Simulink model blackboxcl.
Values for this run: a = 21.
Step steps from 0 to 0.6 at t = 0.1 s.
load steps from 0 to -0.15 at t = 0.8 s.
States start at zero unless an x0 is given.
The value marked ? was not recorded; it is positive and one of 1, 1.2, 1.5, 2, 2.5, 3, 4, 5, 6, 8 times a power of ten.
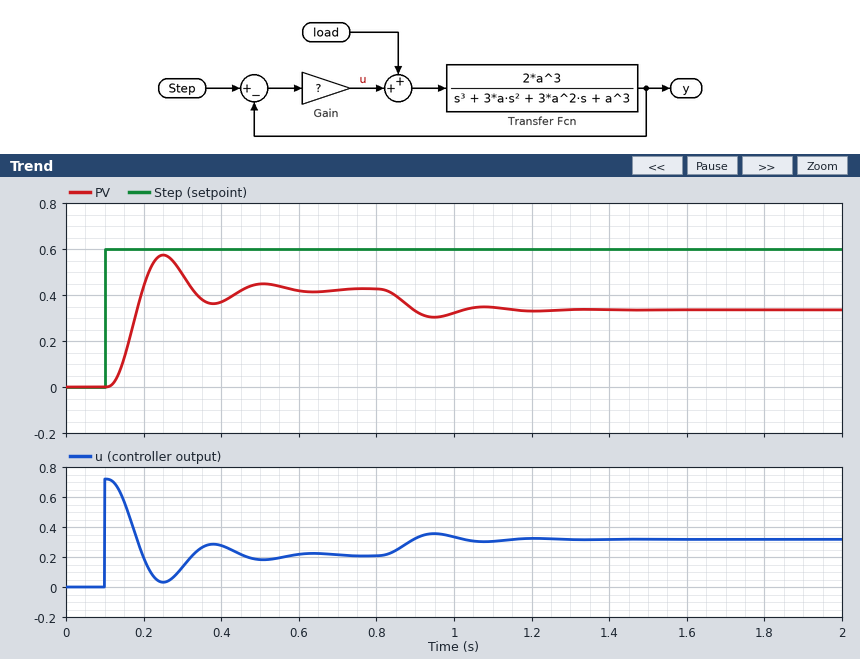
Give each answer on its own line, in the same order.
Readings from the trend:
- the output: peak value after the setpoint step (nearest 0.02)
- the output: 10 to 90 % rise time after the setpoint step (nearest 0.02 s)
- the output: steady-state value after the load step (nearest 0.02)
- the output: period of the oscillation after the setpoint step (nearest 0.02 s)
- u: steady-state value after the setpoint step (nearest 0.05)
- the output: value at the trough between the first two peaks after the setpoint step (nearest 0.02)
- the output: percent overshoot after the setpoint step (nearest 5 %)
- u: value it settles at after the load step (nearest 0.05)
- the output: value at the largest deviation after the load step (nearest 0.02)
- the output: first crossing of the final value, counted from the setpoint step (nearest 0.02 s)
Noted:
0.58
0.06 s
0.34
0.26 s
0.20
0.36
35 %
0.30
0.30
0.10 s
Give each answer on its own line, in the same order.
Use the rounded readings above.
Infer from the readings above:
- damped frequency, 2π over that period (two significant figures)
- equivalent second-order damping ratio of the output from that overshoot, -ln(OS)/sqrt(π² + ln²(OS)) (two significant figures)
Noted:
24 rad/s
0.32
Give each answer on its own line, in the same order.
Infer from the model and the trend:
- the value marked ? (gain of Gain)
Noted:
1.2
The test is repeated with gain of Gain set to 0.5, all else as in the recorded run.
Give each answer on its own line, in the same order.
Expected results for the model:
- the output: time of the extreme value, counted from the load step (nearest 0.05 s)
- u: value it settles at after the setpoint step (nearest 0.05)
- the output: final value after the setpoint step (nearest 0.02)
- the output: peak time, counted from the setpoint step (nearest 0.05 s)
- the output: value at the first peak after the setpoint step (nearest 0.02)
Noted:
0.20 s
0.15
0.30
0.20 s
0.34
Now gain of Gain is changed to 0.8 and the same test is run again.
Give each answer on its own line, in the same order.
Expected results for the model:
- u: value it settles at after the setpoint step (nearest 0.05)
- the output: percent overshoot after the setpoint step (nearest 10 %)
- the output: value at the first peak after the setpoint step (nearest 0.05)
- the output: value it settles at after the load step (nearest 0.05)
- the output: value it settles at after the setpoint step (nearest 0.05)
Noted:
0.20
20 %
0.45
0.25
0.35
